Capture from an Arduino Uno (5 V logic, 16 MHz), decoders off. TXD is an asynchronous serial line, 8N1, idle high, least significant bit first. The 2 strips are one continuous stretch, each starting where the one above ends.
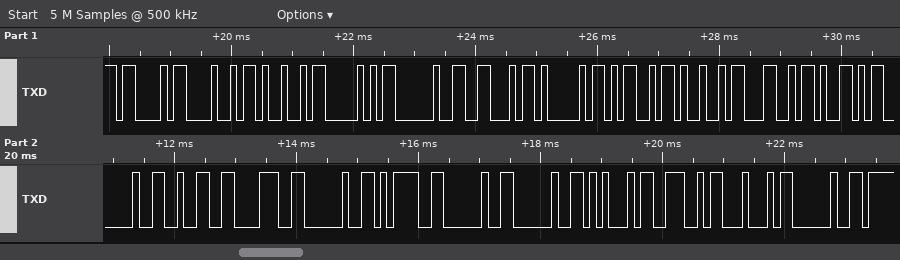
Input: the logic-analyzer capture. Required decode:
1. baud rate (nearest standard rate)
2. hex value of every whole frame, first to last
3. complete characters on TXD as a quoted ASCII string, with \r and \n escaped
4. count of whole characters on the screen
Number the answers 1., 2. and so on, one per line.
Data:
1. 9600 baud
2. 43 48 49 50 20 46 41 4D 49 4C 59 20 32 38 20 3D 20 20 45 4E 44 20
3. "CHIP FAMILY 28 =  END "
4. 22
